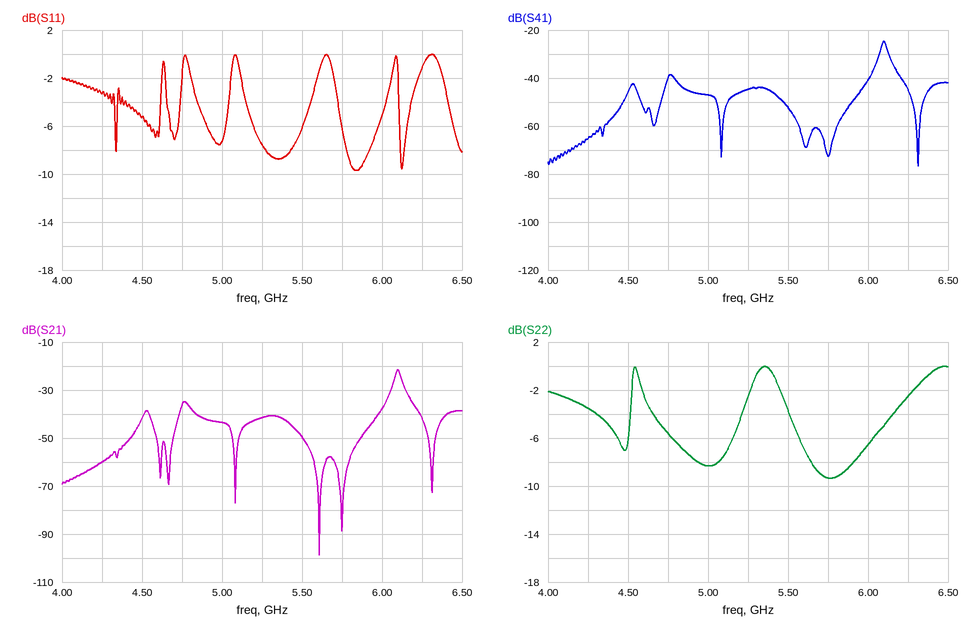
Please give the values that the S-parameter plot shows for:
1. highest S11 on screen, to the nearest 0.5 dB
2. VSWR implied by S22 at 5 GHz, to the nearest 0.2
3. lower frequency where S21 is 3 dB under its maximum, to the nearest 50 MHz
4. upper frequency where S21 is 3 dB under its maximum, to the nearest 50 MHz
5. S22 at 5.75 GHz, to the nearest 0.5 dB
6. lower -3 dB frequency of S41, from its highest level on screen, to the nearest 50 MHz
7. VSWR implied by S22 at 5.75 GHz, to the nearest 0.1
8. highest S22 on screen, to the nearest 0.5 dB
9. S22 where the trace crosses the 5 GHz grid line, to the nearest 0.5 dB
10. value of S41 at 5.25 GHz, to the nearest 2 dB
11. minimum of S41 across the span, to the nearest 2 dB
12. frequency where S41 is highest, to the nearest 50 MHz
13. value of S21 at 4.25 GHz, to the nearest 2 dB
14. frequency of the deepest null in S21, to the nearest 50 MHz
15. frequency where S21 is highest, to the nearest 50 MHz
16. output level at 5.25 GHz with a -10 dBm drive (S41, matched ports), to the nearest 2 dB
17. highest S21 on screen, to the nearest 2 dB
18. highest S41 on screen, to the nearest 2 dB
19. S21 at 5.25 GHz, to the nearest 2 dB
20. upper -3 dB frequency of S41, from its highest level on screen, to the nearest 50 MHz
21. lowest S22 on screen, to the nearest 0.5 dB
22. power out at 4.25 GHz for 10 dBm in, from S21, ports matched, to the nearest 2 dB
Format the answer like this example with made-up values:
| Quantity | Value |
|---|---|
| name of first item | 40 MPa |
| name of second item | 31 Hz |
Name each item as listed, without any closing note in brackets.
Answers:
| Quantity | Value |
|---|---|
| highest S11 on screen, to the nearest 0.5 dB | 0.0 dB |
| VSWR implied by S22 at 5 GHz, to the nearest 0.2 | 2.2 |
| lower frequency where S21 is 3 dB under its maximum, to the nearest 50 MHz | 6.10 GHz |
| upper frequency where S21 is 3 dB under its maximum, to the nearest 50 MHz | 6.10 GHz |
| S22 at 5.75 GHz, to the nearest 0.5 dB | -9.5 dB |
| lower -3 dB frequency of S41, from its highest level on screen, to the nearest 50 MHz | 6.10 GHz |
| VSWR implied by S22 at 5.75 GHz, to the nearest 0.1 | 2.0 |
| highest S22 on screen, to the nearest 0.5 dB | 0.0 dB |
| S22 where the trace crosses the 5 GHz grid line, to the nearest 0.5 dB | -8.5 dB |
| value of S41 at 5.25 GHz, to the nearest 2 dB | -44 dB |
| minimum of S41 across the span, to the nearest 2 dB | -76 dB |
| frequency where S41 is highest, to the nearest 50 MHz | 6.10 GHz |
| value of S21 at 4.25 GHz, to the nearest 2 dB | -60 dB |
| frequency of the deepest null in S21, to the nearest 50 MHz | 5.60 GHz |
| frequency where S21 is highest, to the nearest 50 MHz | 6.10 GHz |
| output level at 5.25 GHz with a -10 dBm drive (S41, matched ports), to the nearest 2 dB | -54 dBm |
| highest S21 on screen, to the nearest 2 dB | -22 dB |
| highest S41 on screen, to the nearest 2 dB | -24 dB |
| S21 at 5.25 GHz, to the nearest 2 dB | -42 dB |
| upper -3 dB frequency of S41, from its highest level on screen, to the nearest 50 MHz | 6.10 GHz |
| lowest S22 on screen, to the nearest 0.5 dB | -9.5 dB |
| power out at 4.25 GHz for 10 dBm in, from S21, ports matched, to the nearest 2 dB | -50 dBm |
